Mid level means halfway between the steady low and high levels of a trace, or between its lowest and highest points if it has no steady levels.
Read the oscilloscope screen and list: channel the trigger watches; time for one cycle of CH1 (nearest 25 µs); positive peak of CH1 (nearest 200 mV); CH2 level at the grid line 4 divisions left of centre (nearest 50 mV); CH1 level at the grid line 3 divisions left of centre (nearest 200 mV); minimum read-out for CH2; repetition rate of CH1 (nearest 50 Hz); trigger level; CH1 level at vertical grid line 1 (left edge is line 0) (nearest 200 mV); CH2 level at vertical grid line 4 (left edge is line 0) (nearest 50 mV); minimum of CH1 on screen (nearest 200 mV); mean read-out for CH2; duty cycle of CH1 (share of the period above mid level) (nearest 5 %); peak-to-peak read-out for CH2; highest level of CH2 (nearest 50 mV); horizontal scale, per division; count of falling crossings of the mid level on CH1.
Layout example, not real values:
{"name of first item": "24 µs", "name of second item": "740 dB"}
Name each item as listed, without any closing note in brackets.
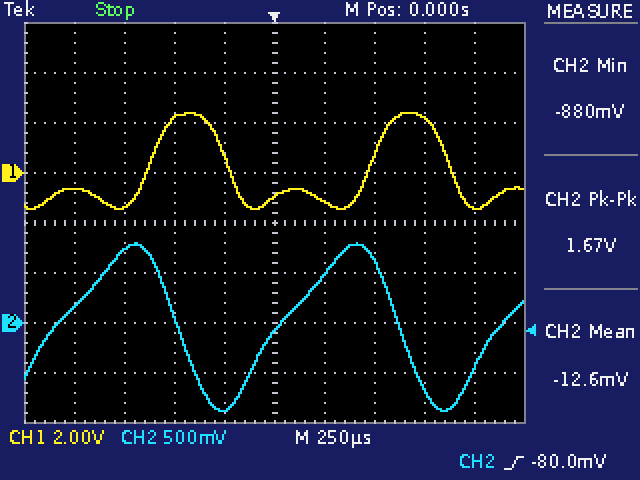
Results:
{"channel the trigger watches": "CH2", "time for one cycle of CH1": "1.100 ms", "positive peak of CH1": "2.4 V", "CH2 level at the grid line 4 divisions left of centre": "150 mV", "CH1 level at the grid line 3 divisions left of centre": "-1.4 V", "minimum read-out for CH2": "-880 mV", "repetition rate of CH1": "900 Hz", "trigger level": "-80.0 mV", "CH1 level at vertical grid line 1 (left edge is line 0)": "-600 mV", "CH2 level at vertical grid line 4 (left edge is line 0)": "-850 mV", "minimum of CH1 on screen": "-1.4 V", "mean read-out for CH2": "-12.6 mV", "duty cycle of CH1 (share of the period above mid level)": "35 %", "peak-to-peak read-out for CH2": "1.67 V", "highest level of CH2": "800 mV", "horizontal scale, per division": "250 µs", "count of falling crossings of the mid level on CH1": "2"}
